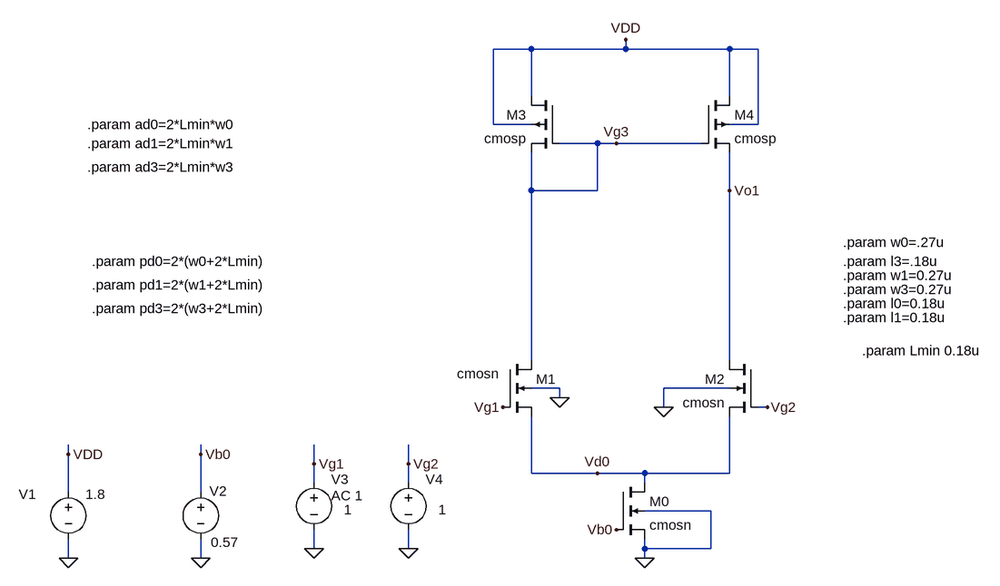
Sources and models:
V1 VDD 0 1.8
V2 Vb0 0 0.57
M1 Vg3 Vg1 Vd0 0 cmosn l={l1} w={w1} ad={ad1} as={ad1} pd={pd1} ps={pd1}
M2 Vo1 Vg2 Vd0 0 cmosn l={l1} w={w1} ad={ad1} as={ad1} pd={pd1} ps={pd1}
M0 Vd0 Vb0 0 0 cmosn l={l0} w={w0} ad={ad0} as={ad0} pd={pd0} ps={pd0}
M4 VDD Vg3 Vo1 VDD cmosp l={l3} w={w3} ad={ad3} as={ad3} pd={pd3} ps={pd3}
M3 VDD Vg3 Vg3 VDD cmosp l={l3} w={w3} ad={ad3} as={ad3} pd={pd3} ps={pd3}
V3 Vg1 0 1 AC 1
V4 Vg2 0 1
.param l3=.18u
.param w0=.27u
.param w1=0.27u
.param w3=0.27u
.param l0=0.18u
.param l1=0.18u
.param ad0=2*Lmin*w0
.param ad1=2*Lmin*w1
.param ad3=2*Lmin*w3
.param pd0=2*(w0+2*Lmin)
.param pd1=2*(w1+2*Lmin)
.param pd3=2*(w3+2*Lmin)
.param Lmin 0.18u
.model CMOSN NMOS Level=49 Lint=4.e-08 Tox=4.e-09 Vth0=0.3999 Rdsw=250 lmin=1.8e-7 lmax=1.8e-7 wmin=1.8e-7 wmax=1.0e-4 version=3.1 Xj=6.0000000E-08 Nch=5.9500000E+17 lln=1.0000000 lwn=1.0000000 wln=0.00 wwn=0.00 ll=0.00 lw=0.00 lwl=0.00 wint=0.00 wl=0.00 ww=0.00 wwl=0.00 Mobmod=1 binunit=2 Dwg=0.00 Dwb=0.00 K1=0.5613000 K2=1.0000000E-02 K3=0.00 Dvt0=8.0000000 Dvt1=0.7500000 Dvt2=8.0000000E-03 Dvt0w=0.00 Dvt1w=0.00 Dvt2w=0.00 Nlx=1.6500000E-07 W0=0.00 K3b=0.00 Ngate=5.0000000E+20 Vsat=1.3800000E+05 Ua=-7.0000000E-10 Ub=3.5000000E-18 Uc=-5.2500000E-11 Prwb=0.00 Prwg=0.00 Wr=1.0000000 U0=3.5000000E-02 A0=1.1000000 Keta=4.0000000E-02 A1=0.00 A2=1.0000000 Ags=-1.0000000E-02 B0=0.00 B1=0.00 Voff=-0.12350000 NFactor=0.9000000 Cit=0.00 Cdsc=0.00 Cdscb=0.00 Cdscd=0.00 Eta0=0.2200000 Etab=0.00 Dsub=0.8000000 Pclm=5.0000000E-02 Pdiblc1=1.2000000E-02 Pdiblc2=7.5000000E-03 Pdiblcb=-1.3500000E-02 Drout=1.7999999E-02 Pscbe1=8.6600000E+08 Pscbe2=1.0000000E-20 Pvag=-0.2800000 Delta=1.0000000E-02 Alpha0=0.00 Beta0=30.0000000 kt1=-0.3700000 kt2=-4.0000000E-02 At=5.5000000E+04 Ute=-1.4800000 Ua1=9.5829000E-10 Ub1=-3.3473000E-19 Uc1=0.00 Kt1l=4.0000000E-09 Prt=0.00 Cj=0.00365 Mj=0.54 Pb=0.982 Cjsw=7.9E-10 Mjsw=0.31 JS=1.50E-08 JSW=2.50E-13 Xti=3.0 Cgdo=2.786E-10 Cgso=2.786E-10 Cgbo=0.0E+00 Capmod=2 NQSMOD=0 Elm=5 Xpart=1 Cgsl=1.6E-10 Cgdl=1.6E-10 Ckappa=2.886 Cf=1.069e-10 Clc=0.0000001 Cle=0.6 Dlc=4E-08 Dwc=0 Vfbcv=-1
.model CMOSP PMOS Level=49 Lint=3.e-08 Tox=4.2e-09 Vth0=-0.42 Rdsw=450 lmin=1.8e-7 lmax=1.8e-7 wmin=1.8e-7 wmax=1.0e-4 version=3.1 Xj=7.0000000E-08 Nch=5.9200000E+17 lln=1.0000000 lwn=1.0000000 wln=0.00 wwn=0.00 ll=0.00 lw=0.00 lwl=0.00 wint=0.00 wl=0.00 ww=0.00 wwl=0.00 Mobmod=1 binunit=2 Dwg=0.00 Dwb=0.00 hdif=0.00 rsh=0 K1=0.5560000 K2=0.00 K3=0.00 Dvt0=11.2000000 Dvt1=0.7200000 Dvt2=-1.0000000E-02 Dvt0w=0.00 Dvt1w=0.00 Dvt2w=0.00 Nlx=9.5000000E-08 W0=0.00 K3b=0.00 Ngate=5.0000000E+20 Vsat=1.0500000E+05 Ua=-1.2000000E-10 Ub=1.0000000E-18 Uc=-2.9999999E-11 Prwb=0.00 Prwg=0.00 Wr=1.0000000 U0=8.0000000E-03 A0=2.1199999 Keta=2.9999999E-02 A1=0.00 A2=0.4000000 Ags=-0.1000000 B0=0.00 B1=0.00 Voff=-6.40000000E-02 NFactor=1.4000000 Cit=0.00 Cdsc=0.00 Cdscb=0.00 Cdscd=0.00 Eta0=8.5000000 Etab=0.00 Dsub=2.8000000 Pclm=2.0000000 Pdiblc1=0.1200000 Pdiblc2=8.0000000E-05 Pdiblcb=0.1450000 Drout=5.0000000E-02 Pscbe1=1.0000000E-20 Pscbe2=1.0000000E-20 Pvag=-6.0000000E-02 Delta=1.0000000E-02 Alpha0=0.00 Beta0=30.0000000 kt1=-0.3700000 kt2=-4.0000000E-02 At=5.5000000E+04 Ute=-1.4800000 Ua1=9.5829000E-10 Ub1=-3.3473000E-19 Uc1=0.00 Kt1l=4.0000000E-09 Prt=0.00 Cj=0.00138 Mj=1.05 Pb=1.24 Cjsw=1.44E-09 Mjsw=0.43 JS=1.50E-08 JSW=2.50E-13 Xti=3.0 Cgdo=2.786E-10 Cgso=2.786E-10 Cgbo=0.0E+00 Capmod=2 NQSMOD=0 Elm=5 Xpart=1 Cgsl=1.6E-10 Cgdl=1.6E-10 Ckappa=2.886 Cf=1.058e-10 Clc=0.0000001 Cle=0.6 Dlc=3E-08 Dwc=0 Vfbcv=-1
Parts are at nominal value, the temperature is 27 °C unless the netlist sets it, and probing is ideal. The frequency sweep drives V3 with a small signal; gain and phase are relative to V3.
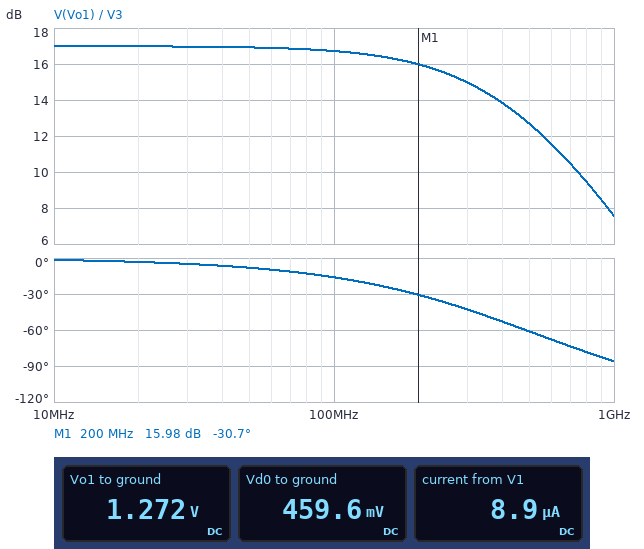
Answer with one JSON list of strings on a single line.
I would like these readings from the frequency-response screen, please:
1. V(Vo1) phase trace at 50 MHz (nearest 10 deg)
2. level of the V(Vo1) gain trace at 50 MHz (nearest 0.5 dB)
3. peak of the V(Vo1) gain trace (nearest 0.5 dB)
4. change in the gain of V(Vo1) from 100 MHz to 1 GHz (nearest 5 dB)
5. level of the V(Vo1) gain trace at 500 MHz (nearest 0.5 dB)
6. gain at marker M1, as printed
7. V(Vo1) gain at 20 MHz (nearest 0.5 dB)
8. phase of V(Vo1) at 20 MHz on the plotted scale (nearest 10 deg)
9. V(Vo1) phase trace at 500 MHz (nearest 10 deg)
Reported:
["-10 deg", "17.0 dB", "17.0 dB", "-10 dB", "12.5 dB", "15.98 dB", "17.0 dB", "0 deg", "-60 deg"]
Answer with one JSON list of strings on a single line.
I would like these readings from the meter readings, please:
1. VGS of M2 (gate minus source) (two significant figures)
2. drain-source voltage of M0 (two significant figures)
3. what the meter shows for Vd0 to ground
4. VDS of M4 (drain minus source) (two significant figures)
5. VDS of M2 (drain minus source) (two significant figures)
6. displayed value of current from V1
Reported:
["540 mV", "460 mV", "459.6 mV", "530 mV", "810 mV", "8.9 µA"]
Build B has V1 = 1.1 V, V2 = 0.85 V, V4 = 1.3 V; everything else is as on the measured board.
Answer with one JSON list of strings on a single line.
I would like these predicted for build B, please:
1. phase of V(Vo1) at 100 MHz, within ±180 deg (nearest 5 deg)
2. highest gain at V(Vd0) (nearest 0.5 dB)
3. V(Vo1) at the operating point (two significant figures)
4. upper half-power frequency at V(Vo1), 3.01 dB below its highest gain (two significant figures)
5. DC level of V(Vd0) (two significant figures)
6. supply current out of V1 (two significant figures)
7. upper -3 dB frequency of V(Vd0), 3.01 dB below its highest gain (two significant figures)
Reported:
["0 deg", "-15.5 dB", "280 mV", "4.3 GHz", "220 mV", "31 µA", "4.1 GHz"]
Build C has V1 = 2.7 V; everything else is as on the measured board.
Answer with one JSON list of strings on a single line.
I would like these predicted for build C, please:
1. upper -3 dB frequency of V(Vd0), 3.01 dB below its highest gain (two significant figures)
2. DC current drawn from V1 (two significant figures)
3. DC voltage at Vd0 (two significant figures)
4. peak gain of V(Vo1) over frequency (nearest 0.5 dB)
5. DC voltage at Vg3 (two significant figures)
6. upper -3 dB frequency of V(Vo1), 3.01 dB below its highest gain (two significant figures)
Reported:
["640 MHz", "9.3 µA", "510 mV", "17.5 dB", "2.2 V", "410 MHz"]
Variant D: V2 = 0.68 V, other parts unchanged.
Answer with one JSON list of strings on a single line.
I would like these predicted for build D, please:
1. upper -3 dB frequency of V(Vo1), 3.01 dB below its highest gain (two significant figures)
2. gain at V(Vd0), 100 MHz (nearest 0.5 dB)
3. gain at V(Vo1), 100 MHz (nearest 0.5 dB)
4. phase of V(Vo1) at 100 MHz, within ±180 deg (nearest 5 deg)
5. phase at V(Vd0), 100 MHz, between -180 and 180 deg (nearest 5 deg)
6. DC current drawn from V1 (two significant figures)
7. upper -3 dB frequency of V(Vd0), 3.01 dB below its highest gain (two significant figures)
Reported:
["630 MHz", "-5.0 dB", "16.0 dB", "-10 deg", "-5 deg", "19 µA", "960 MHz"]
